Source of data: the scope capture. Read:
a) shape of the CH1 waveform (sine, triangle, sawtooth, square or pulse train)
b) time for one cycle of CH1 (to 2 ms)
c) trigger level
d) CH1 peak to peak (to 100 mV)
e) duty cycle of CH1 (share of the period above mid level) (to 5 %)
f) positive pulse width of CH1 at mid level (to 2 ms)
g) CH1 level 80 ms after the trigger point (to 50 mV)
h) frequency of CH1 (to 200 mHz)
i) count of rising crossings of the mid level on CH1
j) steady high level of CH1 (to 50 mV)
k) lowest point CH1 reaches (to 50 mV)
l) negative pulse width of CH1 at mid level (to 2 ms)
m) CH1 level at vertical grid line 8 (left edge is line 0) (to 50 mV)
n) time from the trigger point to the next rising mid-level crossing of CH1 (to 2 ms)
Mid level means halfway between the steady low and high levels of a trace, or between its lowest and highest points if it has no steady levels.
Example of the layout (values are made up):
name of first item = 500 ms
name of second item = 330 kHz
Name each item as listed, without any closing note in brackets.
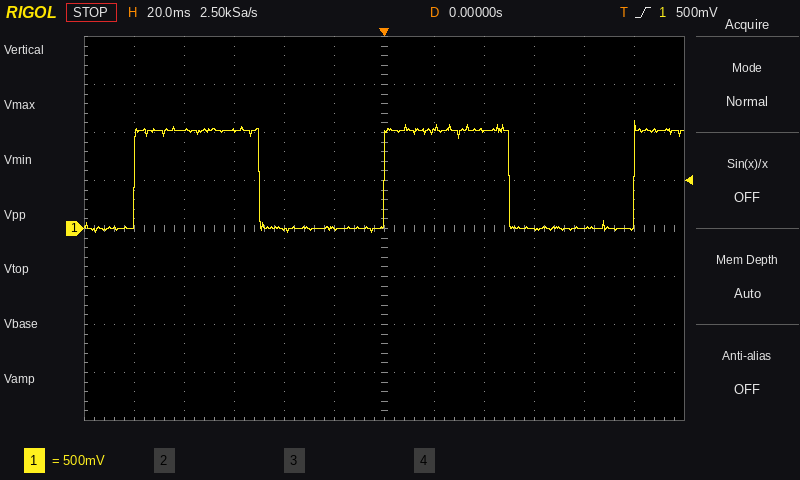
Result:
shape of the CH1 waveform = square
time for one cycle of CH1 = 100 ms
trigger level = 500 mV
CH1 peak to peak = 1.20 V
duty cycle of CH1 (share of the period above mid level) = 50 %
positive pulse width of CH1 at mid level = 50 ms
CH1 level 80 ms after the trigger point = 0 mV
frequency of CH1 = 10.0 Hz
count of rising crossings of the mid level on CH1 = 3
steady high level of CH1 = 1.00 V
lowest point CH1 reaches = -50 mV
negative pulse width of CH1 at mid level = 50 ms
CH1 level at vertical grid line 8 (left edge is line 0) = 1.00 V
time from the trigger point to the next rising mid-level crossing of CH1 = 100 ms
